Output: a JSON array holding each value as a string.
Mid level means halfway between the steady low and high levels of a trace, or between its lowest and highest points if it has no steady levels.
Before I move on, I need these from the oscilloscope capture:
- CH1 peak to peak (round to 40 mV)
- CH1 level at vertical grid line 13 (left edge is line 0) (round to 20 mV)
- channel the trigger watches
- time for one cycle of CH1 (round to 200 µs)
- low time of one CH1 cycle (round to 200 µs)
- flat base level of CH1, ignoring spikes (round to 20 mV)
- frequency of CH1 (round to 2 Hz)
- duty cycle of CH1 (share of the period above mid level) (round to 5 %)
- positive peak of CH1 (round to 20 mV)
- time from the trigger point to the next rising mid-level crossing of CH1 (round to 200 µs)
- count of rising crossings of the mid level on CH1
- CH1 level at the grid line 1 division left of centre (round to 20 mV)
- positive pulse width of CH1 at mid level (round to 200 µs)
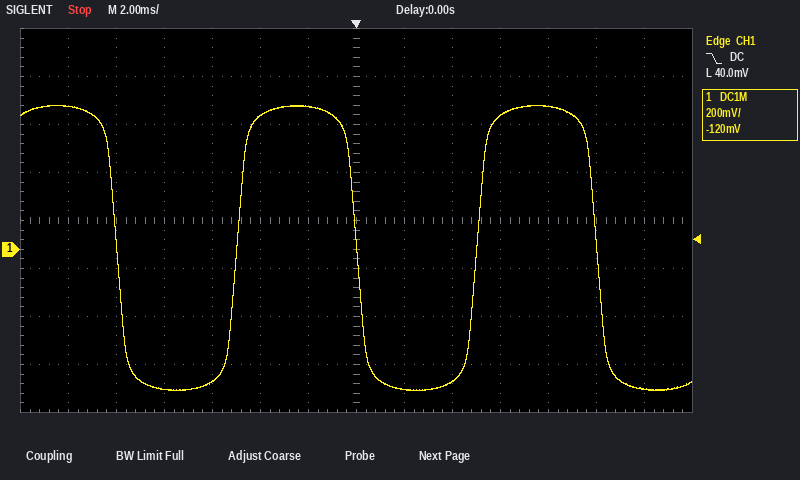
["1.20 V", "-580 mV", "CH1", "10.0 ms", "5.0 ms", "-580 mV", "100 Hz", "50 %", "600 mV", "5.0 ms", "2", "600 mV", "5.0 ms"]
